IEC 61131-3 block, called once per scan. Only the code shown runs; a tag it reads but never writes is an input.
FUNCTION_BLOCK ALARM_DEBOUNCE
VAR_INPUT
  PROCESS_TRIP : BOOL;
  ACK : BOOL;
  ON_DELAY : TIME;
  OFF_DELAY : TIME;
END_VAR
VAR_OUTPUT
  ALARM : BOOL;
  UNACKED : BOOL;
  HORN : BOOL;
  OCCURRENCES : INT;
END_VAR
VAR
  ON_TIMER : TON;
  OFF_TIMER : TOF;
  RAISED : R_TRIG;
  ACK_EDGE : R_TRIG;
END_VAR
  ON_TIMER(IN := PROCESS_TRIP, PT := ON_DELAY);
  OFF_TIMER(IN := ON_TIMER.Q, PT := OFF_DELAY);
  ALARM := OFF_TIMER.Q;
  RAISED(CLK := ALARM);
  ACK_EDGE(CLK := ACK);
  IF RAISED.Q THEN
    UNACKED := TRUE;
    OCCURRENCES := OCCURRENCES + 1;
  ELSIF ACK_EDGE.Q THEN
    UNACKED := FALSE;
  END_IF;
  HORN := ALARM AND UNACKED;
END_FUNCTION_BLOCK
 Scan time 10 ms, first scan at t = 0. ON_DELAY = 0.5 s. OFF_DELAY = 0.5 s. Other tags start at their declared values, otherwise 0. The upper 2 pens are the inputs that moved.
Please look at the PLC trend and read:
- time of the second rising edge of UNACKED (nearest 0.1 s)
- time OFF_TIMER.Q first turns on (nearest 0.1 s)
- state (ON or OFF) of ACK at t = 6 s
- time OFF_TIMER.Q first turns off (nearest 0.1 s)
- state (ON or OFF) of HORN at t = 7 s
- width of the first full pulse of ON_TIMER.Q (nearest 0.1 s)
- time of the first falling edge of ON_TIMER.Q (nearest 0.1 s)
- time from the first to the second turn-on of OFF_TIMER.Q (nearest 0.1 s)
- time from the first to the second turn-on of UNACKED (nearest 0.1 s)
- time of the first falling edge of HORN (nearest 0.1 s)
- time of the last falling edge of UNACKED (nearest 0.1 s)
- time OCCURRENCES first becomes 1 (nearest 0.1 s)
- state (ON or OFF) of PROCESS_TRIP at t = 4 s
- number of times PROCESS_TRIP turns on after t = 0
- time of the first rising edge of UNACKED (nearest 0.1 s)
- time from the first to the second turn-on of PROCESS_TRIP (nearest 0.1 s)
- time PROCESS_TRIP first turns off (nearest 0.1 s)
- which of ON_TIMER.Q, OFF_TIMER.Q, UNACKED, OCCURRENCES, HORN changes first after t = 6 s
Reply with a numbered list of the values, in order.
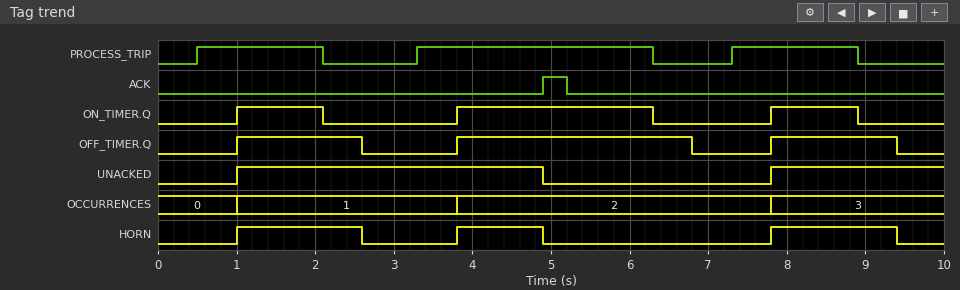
1. 7.8 s
2. 1.0 s
3. OFF
4. 2.6 s
5. OFF
6. 1.1 s
7. 2.1 s
8. 2.8 s
9. 6.8 s
10. 2.6 s
11. 4.9 s
12. 1.0 s
13. ON
14. 3
15. 1.0 s
16. 2.8 s
17. 2.1 s
18. ON_TIMER.Q
